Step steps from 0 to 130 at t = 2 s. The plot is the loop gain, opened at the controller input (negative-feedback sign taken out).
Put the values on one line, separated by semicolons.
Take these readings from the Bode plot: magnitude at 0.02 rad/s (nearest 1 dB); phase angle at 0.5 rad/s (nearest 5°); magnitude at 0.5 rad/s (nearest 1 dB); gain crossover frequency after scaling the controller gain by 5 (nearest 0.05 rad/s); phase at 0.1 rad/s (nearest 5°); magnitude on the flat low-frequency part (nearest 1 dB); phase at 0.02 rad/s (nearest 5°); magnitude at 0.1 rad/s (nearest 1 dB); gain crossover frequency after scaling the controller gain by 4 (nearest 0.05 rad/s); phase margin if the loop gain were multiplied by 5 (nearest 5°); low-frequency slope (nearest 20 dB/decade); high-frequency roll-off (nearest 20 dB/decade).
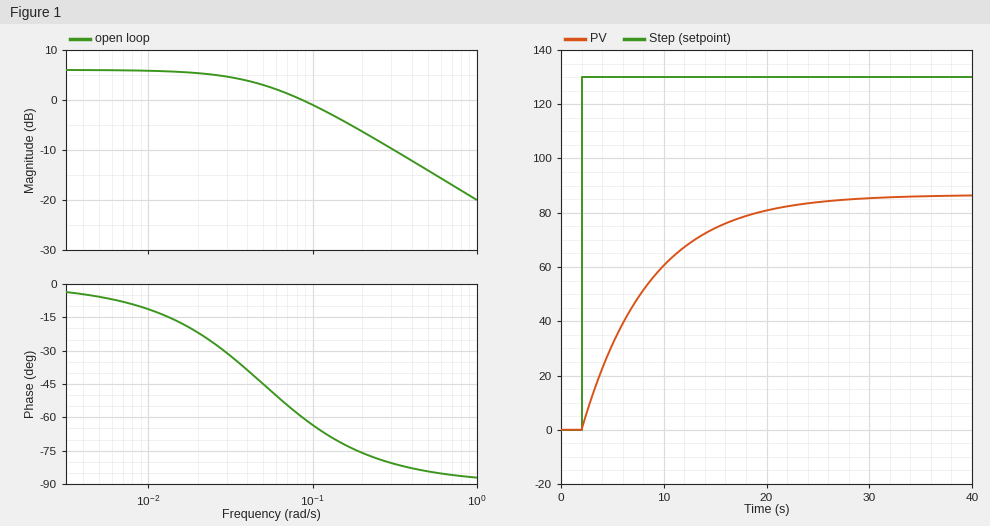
5 dB; -85°; -14 dB; 0.50 rad/s; -65°; 6 dB; -20°; -1 dB; 0.40 rad/s; 95°; 0 dB/decade; -20 dB/decade
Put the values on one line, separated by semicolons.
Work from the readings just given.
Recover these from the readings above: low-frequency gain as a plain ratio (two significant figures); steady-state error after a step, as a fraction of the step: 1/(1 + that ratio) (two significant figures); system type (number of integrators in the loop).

2.0; 0.33; 0
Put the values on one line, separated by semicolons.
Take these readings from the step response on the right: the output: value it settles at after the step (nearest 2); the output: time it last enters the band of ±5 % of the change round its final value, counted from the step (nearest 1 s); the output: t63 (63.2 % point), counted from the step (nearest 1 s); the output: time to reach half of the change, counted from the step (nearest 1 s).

86; 20 s; 7 s; 5 s
